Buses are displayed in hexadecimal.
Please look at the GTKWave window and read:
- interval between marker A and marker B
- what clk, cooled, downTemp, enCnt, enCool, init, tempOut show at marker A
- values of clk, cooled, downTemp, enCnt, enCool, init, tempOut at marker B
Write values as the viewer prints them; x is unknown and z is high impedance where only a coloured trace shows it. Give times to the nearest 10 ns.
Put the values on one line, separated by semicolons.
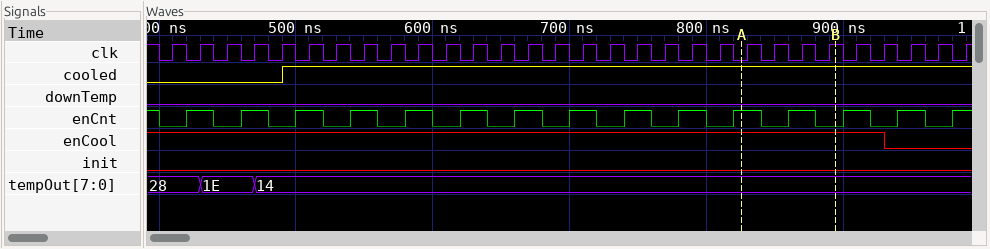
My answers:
70 ns; clk=0, cooled=1, downTemp=0, enCnt=1, enCool=1, init=0, tempOut=14; clk=1, cooled=1, downTemp=0, enCnt=0, enCool=1, init=0, tempOut=14
